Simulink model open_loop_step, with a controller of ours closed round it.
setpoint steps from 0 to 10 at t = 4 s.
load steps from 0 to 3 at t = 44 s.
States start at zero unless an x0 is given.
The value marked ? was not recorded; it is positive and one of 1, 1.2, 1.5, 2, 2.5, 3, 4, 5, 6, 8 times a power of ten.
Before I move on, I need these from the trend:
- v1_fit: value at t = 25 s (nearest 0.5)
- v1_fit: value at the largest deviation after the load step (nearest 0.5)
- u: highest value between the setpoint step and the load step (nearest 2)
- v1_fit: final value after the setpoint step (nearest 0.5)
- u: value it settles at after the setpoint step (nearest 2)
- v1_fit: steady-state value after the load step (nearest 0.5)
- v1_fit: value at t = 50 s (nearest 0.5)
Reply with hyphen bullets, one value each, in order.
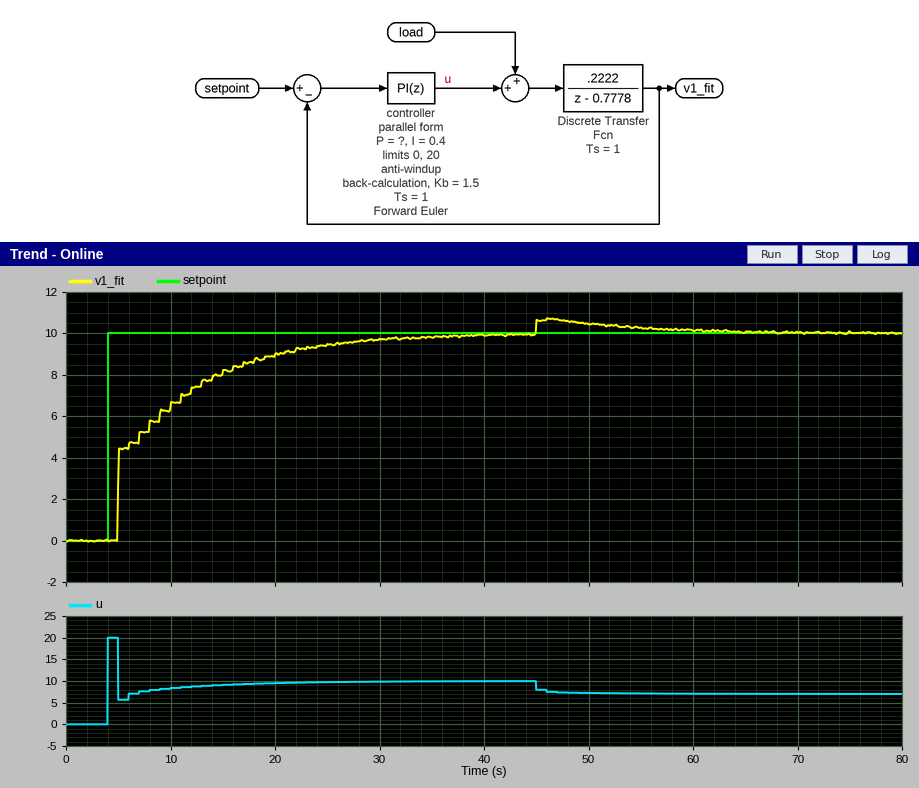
- 9.5
- 10.5
- 20
- 10.0
- 10
- 10.0
- 10.5
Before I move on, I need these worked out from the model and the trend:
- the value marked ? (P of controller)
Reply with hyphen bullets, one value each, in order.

- 3
